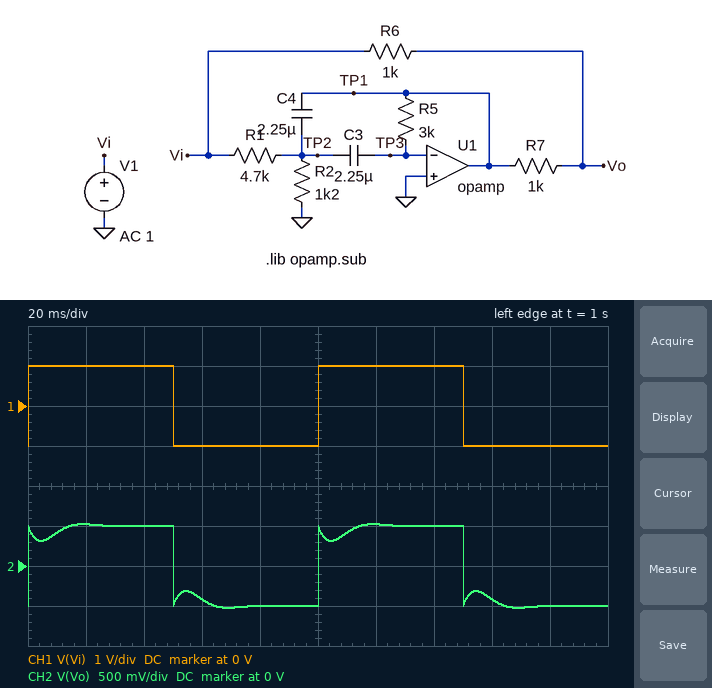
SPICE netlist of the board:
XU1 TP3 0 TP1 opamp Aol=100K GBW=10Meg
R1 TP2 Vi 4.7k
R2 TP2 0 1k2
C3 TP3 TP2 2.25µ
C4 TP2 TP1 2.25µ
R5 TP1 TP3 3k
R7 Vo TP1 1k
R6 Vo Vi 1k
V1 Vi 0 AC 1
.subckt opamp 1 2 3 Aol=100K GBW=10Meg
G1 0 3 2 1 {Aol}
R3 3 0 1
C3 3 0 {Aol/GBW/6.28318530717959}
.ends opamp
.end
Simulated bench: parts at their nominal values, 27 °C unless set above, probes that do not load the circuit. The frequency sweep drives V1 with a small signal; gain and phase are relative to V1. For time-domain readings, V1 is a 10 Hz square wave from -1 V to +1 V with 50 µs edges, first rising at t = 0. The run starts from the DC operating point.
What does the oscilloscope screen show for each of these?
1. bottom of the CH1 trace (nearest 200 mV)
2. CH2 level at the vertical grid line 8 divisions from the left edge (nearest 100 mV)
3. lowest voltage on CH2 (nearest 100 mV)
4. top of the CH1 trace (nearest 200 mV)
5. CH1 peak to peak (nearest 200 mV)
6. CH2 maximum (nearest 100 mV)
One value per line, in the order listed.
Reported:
-1.0 V
-400 mV
-500 mV
1.0 V
2.0 V
500 mV
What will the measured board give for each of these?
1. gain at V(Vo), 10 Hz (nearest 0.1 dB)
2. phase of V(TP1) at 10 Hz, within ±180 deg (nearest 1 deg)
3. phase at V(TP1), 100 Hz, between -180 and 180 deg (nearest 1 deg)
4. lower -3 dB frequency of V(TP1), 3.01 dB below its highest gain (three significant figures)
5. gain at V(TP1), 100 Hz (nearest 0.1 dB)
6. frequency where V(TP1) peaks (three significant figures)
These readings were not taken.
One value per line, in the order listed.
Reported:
-6.2 dB
-106 deg
120 deg
24.4 Hz
-16.0 dB
41.8 Hz
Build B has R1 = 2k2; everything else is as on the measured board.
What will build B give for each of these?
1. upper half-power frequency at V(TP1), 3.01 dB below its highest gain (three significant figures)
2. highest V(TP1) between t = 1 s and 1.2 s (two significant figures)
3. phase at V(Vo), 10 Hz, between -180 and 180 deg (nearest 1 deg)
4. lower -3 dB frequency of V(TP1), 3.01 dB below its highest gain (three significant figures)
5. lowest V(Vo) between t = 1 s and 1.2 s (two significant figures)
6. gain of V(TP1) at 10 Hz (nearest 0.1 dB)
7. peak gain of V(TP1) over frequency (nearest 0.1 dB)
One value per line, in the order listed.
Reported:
75.6 Hz
750 mV
-9 deg
28.4 Hz
-560 mV
-16.3 dB
-3.3 dB
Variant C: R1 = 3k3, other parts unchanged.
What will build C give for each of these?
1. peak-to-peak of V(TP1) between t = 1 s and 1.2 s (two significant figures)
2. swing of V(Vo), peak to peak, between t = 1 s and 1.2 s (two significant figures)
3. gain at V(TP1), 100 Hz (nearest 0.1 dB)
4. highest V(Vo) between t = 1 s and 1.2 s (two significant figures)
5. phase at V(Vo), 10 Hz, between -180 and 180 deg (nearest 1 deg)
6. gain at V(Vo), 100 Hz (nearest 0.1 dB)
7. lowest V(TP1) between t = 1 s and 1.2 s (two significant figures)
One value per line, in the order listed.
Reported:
1.0 V
1.1 V
-12.8 dB
530 mV
-7 deg
-6.9 dB
-520 mV
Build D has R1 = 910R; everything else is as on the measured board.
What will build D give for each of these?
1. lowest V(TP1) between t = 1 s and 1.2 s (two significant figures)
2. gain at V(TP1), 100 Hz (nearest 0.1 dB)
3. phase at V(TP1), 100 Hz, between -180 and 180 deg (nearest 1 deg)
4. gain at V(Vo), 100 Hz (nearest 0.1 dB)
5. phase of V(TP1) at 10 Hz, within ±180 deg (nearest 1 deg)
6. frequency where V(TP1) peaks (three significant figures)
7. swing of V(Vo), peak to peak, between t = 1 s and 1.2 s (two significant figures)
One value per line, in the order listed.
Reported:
-1.6 V
-0.5 dB
125 deg
-6.9 dB
-99 deg
56.8 Hz
1.4 V
